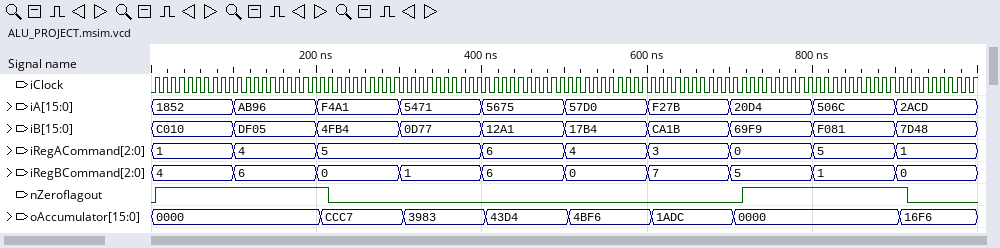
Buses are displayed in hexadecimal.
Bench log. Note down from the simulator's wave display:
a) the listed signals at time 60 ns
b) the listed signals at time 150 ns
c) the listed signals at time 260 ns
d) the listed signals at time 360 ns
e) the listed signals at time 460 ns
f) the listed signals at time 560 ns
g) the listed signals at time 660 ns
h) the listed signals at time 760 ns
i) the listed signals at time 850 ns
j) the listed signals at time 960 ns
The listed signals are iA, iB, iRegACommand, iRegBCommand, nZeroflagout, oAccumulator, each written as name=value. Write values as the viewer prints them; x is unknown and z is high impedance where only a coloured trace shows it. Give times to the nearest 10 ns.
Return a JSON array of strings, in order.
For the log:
["iA=1852, iB=C010, iRegACommand=1, iRegBCommand=4, nZeroflagout=1, oAccumulator=0000", "iA=AB96, iB=DF05, iRegACommand=4, iRegBCommand=6, nZeroflagout=1, oAccumulator=0000", "iA=F4A1, iB=4FB4, iRegACommand=5, iRegBCommand=0, nZeroflagout=0, oAccumulator=CCC7", "iA=5471, iB=0D77, iRegACommand=5, iRegBCommand=1, nZeroflagout=0, oAccumulator=3983", "iA=5675, iB=12A1, iRegACommand=6, iRegBCommand=6, nZeroflagout=0, oAccumulator=43D4", "iA=57D0, iB=17B4, iRegACommand=4, iRegBCommand=0, nZeroflagout=0, oAccumulator=4BF6", "iA=F27B, iB=CA1B, iRegACommand=3, iRegBCommand=7, nZeroflagout=0, oAccumulator=1ADC", "iA=20D4, iB=69F9, iRegACommand=0, iRegBCommand=5, nZeroflagout=1, oAccumulator=0000", "iA=506C, iB=F081, iRegACommand=5, iRegBCommand=1, nZeroflagout=1, oAccumulator=0000", "iA=2ACD, iB=7D48, iRegACommand=1, iRegBCommand=0, nZeroflagout=0, oAccumulator=16F6"]
